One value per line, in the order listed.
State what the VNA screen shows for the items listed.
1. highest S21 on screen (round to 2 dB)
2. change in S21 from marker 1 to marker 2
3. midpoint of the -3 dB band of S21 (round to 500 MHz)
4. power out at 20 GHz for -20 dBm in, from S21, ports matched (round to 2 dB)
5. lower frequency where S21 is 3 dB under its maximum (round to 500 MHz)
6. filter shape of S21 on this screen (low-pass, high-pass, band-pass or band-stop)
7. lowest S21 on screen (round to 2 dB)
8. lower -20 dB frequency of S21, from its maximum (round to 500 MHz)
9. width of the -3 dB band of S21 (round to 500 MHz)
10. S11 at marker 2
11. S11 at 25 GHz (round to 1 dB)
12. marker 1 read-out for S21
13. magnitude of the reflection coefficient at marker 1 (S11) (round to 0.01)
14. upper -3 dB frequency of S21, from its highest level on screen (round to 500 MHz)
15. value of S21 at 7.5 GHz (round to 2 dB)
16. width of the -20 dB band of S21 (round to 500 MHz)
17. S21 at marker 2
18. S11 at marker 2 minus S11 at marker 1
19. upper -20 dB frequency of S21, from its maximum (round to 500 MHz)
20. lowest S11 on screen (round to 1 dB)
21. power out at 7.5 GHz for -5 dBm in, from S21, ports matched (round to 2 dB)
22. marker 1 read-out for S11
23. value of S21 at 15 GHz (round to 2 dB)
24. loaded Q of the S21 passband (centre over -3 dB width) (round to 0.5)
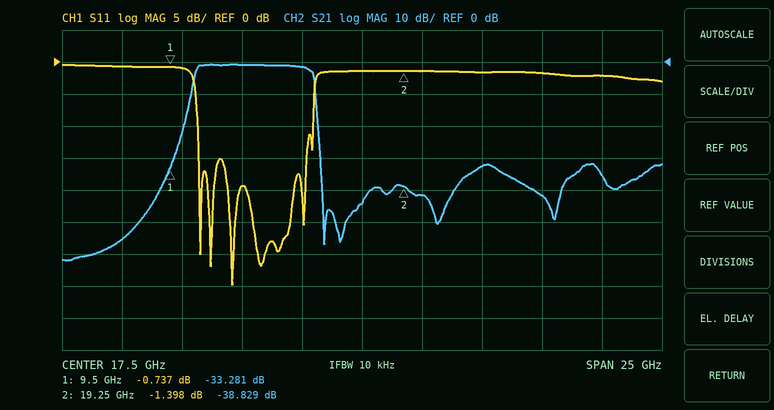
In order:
0 dB
-5.548 dB
13.0 GHz
-62 dBm
10.5 GHz
band-pass
-62 dB
10.0 GHz
5.0 GHz
-1.398 dB
-2 dB
-33.281 dB
0.92
15.5 GHz
-56 dB
5.5 GHz
-38.829 dB
-0.661 dB
15.5 GHz
-35 dB
-60 dBm
-0.737 dB
-2 dB
2.5
